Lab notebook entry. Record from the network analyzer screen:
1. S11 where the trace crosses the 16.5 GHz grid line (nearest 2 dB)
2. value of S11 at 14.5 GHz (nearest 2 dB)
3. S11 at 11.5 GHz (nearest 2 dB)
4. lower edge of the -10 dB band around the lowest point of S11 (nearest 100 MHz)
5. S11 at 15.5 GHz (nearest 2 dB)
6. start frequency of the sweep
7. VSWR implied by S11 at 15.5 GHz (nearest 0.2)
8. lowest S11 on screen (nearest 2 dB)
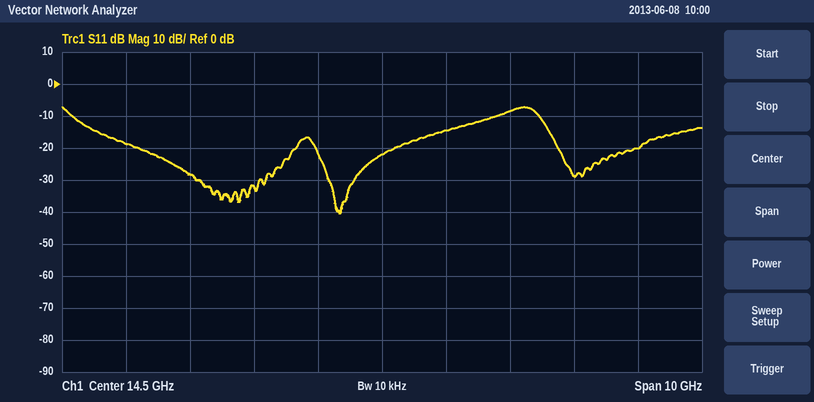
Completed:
-8 dB
-22 dB
-28 dB
9.7 GHz
-14 dB
9.5 GHz
1.4
-40 dB
